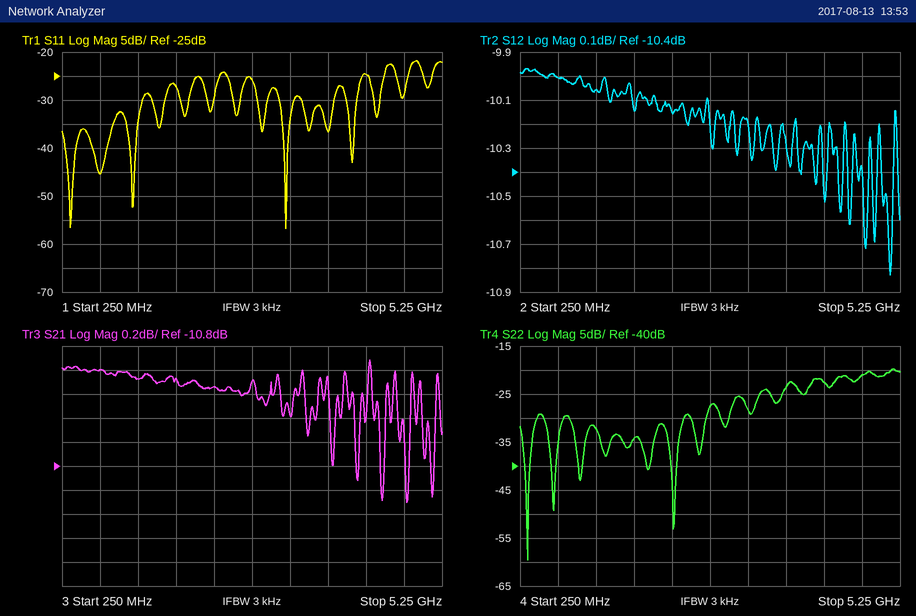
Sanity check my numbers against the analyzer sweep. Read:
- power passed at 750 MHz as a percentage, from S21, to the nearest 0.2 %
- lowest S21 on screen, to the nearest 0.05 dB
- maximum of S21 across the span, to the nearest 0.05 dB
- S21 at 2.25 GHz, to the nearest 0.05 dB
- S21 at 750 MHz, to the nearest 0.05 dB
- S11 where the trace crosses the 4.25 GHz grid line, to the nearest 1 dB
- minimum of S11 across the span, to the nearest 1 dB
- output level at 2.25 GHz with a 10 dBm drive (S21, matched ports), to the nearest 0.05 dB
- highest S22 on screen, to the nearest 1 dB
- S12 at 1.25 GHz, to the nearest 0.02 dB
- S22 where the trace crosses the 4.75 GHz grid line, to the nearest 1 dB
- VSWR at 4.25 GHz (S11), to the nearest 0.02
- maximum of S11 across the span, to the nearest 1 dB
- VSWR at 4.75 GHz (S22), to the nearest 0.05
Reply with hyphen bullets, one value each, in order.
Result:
- 10.0 %
- -11.10 dB
- -9.90 dB
- -10.15 dB
- -10.00 dB
- -25 dB
- -57 dB
- -0.15 dBm
- -20 dB
- -10.06 dB
- -21 dB
- 1.12
- -22 dB
- 1.20
